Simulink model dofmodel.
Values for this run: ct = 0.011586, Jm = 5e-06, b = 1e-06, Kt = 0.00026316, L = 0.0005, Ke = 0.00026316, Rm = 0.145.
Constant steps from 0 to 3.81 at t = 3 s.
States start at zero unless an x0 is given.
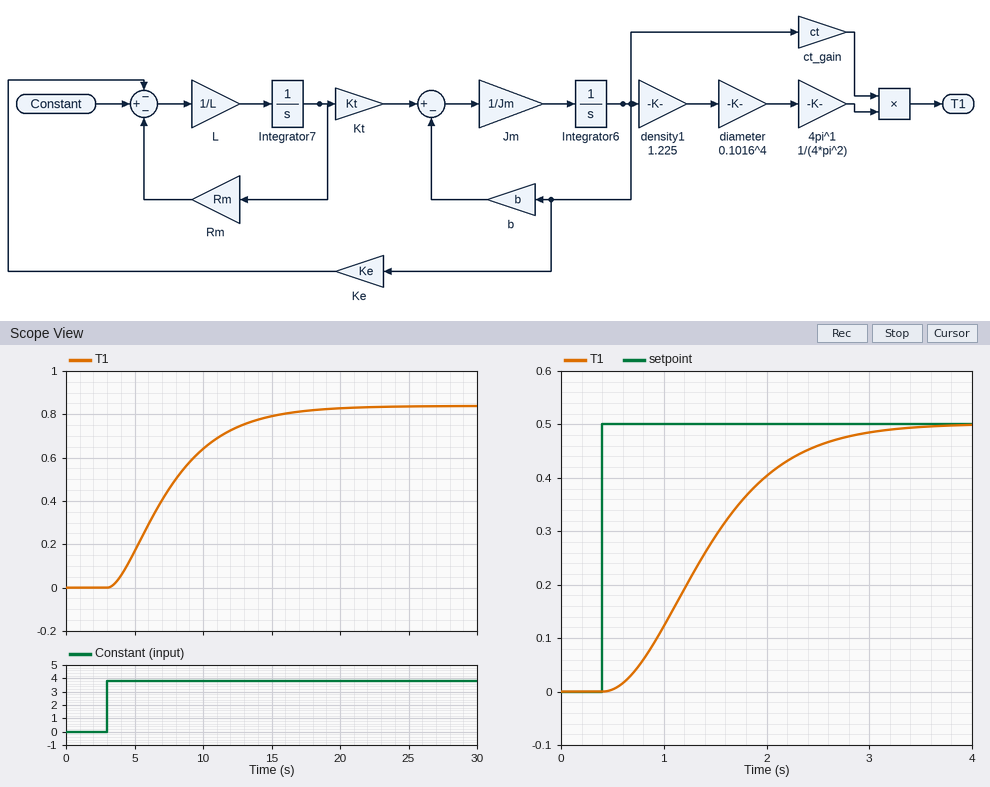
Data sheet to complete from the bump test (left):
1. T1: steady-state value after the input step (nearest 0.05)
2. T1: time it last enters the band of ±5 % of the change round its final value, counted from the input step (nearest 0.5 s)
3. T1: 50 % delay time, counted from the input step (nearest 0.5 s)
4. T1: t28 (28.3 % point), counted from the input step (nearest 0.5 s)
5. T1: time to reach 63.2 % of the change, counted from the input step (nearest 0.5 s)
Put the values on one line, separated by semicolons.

0.85; 12.5 s; 4.0 s; 2.5 s; 5.5 s
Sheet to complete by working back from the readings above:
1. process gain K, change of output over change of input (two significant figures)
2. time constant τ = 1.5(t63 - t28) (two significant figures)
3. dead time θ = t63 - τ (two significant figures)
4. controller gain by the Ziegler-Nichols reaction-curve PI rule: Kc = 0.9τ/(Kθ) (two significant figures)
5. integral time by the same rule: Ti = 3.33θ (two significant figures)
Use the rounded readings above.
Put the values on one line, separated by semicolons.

0.22; 4.5 s; 1.0 s; 18; 3.3 s
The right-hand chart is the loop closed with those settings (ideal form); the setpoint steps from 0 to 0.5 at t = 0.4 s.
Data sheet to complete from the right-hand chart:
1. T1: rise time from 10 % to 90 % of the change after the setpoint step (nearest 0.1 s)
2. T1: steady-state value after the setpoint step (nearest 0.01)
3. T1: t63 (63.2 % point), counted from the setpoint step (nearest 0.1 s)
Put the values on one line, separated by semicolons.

1.6 s; 0.50; 1.2 s
